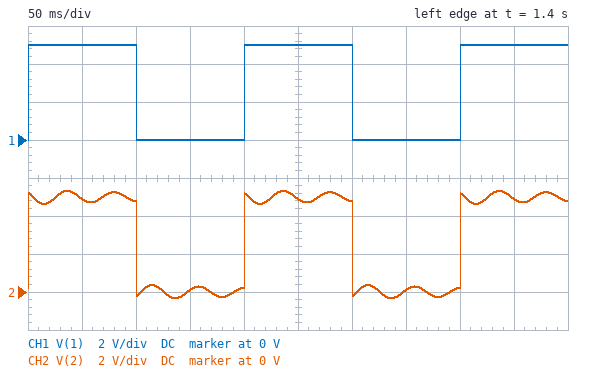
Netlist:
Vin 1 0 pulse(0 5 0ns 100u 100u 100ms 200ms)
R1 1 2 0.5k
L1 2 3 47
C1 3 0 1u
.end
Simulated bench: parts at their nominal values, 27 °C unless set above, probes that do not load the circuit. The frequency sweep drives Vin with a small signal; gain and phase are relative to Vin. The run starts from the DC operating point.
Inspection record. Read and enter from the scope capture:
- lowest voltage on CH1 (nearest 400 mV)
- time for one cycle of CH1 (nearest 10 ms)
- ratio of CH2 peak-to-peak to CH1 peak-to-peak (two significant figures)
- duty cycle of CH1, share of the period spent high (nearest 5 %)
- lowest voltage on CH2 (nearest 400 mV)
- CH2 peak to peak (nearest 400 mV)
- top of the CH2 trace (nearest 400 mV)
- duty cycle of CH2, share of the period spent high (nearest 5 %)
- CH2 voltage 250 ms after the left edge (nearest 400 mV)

0 V
200 ms
1.1
50 %
-400 mV
5.6 V
5.2 V
50 %
4.8 V
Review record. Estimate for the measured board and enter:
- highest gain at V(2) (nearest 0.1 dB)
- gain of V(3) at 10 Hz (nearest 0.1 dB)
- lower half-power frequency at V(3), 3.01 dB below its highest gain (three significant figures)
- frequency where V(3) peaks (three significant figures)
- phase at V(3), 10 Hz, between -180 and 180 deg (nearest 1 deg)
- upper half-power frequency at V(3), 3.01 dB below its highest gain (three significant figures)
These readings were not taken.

0 dB
1.8 dB
22.3 Hz
23.2 Hz
-2 deg
24.0 Hz
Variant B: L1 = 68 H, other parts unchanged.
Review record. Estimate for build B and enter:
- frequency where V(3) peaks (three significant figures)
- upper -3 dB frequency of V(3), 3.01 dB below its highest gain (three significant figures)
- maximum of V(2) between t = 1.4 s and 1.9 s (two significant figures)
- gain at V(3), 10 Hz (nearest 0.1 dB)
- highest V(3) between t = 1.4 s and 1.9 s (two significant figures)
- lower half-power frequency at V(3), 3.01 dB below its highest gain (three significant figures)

19.3 Hz
19.9 Hz
5.2 V
2.7 dB
7.8 V
18.7 Hz
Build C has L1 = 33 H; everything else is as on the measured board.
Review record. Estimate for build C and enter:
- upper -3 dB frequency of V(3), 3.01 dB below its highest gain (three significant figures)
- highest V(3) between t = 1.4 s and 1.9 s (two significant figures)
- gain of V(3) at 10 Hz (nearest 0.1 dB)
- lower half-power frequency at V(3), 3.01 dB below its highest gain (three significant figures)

28.8 Hz
8.9 V
1.2 dB
26.4 Hz
